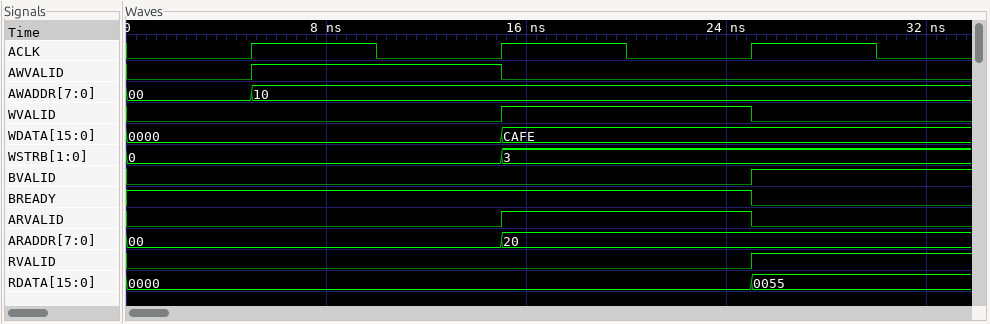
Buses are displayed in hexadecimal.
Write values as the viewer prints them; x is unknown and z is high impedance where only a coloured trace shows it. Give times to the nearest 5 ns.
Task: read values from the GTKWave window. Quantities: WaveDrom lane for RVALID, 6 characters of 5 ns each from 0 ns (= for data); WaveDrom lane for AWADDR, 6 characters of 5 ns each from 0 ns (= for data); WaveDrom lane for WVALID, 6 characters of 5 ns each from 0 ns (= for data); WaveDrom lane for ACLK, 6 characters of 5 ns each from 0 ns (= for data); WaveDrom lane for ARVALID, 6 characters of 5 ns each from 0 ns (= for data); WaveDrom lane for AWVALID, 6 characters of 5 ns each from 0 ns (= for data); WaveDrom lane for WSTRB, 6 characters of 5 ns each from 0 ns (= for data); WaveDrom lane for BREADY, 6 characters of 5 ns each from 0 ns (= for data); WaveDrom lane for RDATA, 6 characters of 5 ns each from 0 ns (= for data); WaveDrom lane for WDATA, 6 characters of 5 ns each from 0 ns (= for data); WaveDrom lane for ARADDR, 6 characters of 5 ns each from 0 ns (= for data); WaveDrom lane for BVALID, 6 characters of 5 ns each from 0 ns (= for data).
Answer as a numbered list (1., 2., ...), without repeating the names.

1. {name: 'RVALID', wave: '0....1'}
2. {name: 'AWADDR', wave: '==....', data: '00 10'}
3. {name: 'WVALID', wave: '0..1.0'}
4. {name: 'ACLK', wave: '010101'}
5. {name: 'ARVALID', wave: '0..1.0'}
6. {name: 'AWVALID', wave: '01.0..'}
7. {name: 'WSTRB', wave: '=..=..', data: '0 3'}
8. {name: 'BREADY', wave: '1....0'}
9. {name: 'RDATA', wave: '=....=', data: '0000 0055'}
10. {name: 'WDATA', wave: '=..=..', data: '0000 CAFE'}
11. {name: 'ARADDR', wave: '=..=..', data: '00 20'}
12. {name: 'BVALID', wave: '0....1'}
